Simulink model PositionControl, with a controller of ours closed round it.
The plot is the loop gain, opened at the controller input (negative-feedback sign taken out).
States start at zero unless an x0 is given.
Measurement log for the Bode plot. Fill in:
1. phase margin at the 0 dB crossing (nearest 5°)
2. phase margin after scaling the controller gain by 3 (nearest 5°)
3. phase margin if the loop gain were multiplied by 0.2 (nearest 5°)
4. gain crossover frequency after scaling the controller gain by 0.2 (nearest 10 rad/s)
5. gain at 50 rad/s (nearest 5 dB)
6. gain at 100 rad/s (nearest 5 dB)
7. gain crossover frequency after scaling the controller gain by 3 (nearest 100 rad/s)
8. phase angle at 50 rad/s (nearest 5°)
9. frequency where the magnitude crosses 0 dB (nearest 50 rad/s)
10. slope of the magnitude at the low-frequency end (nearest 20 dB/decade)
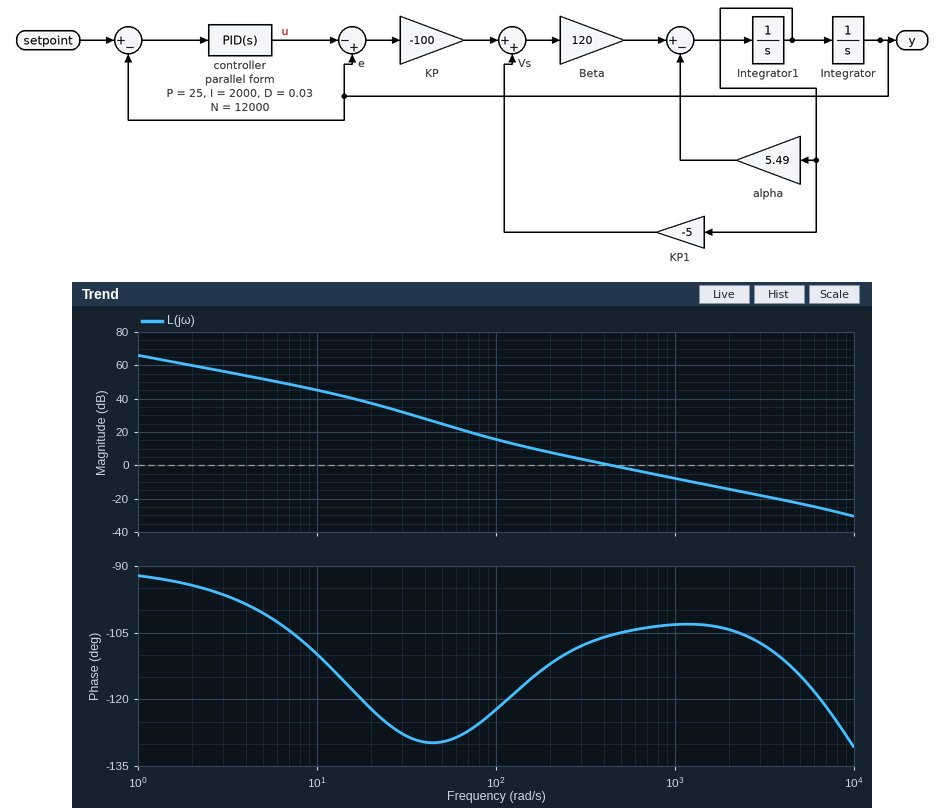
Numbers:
75°
75°
60°
110 rad/s
25 dB
15 dB
1200 rad/s
-130°
450 rad/s
-20 dB/decade
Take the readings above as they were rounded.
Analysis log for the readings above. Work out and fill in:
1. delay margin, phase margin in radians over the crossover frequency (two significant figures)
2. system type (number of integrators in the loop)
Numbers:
0.0029 s
1
